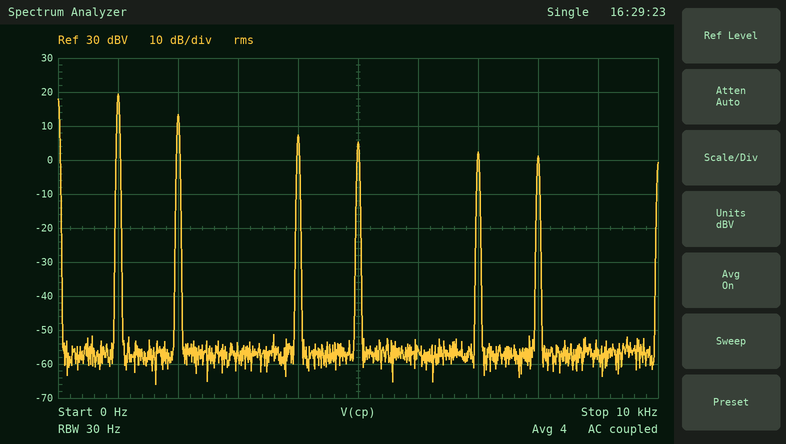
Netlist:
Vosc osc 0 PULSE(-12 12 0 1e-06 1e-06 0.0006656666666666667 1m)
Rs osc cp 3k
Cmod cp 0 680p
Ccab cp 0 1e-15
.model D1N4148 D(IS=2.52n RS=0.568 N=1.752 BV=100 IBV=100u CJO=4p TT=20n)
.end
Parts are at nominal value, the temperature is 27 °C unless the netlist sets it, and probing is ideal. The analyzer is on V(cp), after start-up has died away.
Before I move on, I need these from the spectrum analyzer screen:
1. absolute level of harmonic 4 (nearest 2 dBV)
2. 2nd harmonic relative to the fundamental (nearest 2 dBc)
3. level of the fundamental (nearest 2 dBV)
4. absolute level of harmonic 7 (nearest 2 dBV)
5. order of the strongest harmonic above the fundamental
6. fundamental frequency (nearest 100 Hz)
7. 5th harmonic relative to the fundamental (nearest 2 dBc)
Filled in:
8 dBV
-6 dBc
20 dBV
2 dBV
2
1.0 kHz
-14 dBc
